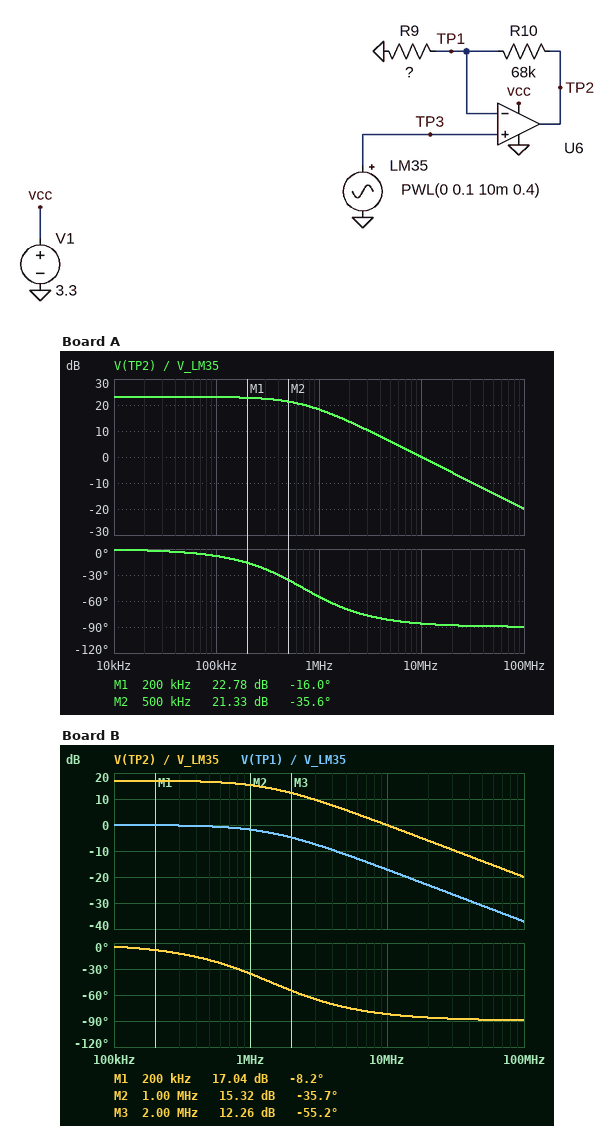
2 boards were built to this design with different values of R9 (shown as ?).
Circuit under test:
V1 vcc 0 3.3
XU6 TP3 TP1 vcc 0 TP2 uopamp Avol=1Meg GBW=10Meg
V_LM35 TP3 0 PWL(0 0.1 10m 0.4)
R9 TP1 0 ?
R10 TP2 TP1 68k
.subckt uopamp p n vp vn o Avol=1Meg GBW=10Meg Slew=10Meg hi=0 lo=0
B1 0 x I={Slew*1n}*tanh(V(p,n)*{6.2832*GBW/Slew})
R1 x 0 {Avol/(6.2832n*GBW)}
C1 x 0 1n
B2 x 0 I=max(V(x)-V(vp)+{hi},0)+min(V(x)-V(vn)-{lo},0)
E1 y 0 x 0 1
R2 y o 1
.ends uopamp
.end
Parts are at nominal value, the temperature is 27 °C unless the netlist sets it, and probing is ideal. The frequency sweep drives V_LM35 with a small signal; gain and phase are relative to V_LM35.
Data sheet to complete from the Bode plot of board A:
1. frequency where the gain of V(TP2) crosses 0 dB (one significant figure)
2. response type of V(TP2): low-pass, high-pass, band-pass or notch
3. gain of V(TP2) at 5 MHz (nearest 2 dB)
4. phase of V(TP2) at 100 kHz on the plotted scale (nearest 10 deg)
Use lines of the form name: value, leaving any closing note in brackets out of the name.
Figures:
frequency where the gain of V(TP2) crosses 0 dB: 10 MHz
response type of V(TP2): low-pass, high-pass, band-pass or notch: low-pass
gain of V(TP2) at 5 MHz: 6 dB
phase of V(TP2) at 100 kHz on the plotted scale: -10 deg
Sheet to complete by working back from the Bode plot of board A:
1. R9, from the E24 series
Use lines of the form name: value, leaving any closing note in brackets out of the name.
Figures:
R9, from the E24 series: 5.1 kΩ
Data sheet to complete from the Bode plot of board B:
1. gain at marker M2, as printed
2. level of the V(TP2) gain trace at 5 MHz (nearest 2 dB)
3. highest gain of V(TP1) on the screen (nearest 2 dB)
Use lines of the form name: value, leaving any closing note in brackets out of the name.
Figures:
gain at marker M2, as printed: 15.32 dB
level of the V(TP2) gain trace at 5 MHz: 6 dB
highest gain of V(TP1) on the screen: 0 dB
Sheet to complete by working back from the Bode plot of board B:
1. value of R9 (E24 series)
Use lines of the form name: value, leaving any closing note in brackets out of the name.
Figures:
value of R9: 11 kΩ
